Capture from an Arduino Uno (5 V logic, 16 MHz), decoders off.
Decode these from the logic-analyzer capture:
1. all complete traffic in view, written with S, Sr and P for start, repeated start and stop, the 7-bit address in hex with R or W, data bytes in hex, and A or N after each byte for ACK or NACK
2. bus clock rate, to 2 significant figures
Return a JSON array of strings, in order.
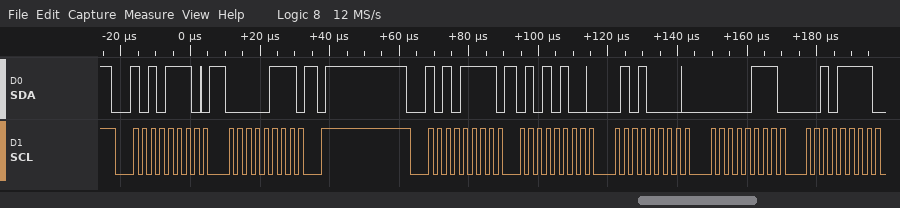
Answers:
["S 57W A 07 A P S 57R A 54 A 50 A 07 A 2F A", "400 kHz"]
